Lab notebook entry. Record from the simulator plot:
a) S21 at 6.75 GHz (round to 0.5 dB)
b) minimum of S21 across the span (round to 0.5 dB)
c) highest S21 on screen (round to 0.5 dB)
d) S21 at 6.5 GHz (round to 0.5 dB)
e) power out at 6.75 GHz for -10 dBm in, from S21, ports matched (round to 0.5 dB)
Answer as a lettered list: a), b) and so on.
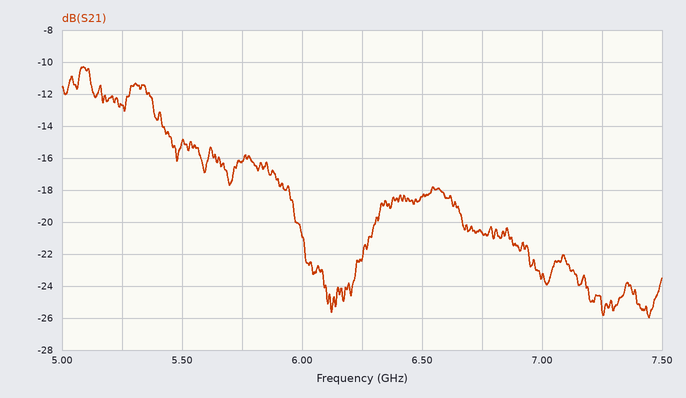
a) -20.5 dB
b) -26.0 dB
c) -10.5 dB
d) -18.5 dB
e) -30.5 dBm
